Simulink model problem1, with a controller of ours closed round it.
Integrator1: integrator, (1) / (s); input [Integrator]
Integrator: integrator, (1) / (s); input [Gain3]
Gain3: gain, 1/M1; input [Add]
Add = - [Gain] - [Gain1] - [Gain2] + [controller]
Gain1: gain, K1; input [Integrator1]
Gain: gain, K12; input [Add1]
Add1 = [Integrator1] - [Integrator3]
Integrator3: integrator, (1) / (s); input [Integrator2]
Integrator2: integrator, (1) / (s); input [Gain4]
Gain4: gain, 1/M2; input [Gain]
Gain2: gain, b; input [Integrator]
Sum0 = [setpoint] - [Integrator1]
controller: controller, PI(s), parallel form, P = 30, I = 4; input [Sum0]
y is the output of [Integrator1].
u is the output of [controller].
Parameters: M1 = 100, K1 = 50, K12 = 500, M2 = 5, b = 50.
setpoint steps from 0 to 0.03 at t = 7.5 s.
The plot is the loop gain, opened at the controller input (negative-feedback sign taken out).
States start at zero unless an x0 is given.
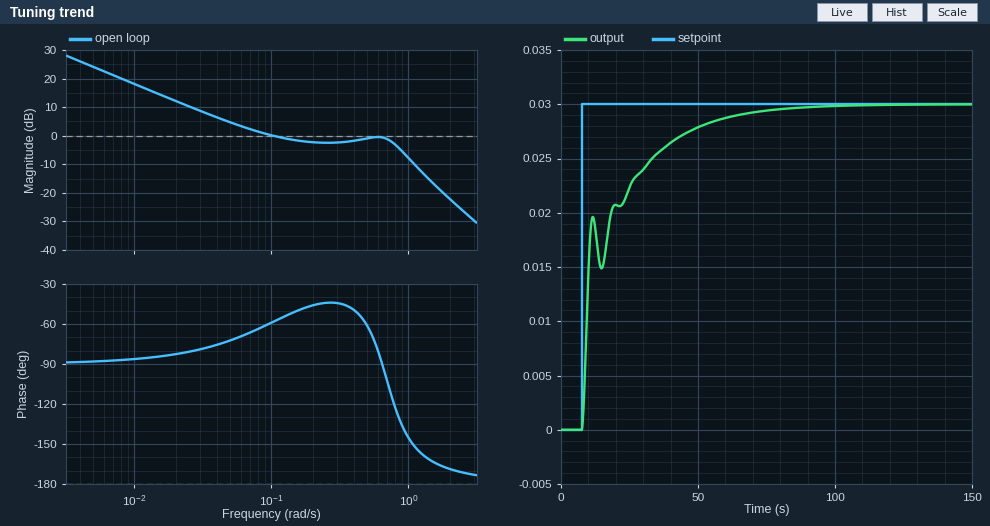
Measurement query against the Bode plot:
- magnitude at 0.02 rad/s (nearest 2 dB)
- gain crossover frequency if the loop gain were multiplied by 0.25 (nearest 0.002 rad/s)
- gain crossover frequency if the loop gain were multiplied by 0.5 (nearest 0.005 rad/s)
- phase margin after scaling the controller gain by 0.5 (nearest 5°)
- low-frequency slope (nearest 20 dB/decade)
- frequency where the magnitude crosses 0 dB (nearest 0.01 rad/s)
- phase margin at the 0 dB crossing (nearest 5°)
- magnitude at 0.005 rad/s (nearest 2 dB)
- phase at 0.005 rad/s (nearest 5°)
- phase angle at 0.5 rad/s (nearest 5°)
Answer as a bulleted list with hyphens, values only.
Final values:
- 12 dB
- 0.020 rad/s
- 0.040 rad/s
- 105°
- -20 dB/decade
- 0.10 rad/s
- 120°
- 24 dB
- -90°
- -60°
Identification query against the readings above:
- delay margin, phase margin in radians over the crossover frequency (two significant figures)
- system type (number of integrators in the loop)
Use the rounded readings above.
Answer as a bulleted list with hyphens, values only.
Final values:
- 21 s
- 1
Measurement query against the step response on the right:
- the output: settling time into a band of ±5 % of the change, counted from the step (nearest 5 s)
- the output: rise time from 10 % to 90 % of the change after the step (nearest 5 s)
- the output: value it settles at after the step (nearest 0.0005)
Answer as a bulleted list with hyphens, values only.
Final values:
- 50 s
- 35 s
- 0.0300
